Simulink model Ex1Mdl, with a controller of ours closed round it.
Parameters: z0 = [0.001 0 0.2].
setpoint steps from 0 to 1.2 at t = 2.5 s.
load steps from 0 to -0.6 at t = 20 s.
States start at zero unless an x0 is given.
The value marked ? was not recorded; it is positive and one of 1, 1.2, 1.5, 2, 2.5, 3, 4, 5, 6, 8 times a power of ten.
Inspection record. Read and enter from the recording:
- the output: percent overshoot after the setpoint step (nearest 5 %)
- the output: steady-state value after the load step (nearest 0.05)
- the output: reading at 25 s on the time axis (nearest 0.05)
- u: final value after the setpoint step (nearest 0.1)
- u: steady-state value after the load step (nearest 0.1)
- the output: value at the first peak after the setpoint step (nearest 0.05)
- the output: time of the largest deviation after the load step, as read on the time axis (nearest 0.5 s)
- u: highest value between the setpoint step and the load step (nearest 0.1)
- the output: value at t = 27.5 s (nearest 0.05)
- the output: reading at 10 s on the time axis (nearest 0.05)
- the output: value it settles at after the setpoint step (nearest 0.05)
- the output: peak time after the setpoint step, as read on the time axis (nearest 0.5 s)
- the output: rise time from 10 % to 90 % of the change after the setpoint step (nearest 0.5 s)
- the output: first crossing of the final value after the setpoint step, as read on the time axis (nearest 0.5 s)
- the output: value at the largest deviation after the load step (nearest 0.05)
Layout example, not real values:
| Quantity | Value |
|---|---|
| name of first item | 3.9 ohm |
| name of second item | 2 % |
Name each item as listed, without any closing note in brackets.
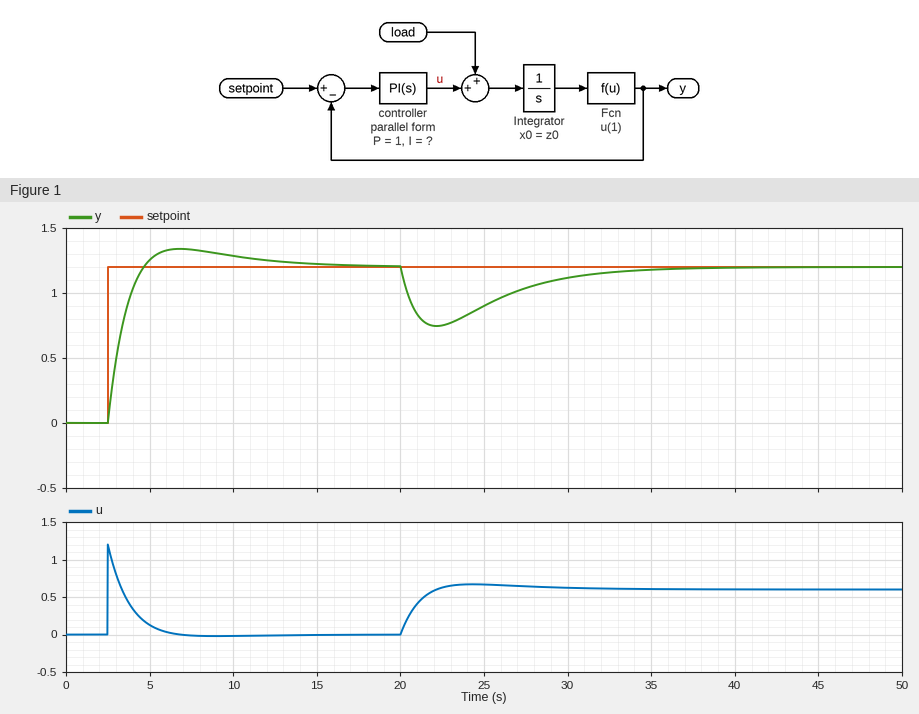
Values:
| Quantity | Value |
|---|---|
| the output: percent overshoot after the setpoint step | 10 % |
| the output: steady-state value after the load step | 1.20 |
| the output: reading at 25 s on the time axis | 0.90 |
| u: final value after the setpoint step | 0.0 |
| u: steady-state value after the load step | 0.6 |
| the output: value at the first peak after the setpoint step | 1.35 |
| the output: time of the largest deviation after the load step, as read on the time axis | 22.0 s |
| u: highest value between the setpoint step and the load step | 1.2 |
| the output: value at t = 27.5 s | 1.05 |
| the output: reading at 10 s on the time axis | 1.30 |
| the output: value it settles at after the setpoint step | 1.20 |
| the output: peak time after the setpoint step, as read on the time axis | 7.0 s |
| the output: rise time from 10 % to 90 % of the change after the setpoint step | 1.5 s |
| the output: first crossing of the final value after the setpoint step, as read on the time axis | 4.5 s |
| the output: value at the largest deviation after the load step | 0.75 |
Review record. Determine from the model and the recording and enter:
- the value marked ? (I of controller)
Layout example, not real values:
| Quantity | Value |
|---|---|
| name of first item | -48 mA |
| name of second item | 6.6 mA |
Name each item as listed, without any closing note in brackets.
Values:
| Quantity | Value |
|---|---|
| the value marked ? | 0.2 |
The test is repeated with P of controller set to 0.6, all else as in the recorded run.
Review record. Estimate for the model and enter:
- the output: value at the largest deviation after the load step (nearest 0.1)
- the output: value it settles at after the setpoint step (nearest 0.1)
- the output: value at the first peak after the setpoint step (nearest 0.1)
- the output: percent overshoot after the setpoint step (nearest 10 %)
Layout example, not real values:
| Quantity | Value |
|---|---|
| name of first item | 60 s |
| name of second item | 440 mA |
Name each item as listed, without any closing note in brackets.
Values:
| Quantity | Value |
|---|---|
| the output: value at the largest deviation after the load step | 0.6 |
| the output: value it settles at after the setpoint step | 1.2 |
| the output: value at the first peak after the setpoint step | 1.5 |
| the output: percent overshoot after the setpoint step | 20 % |
